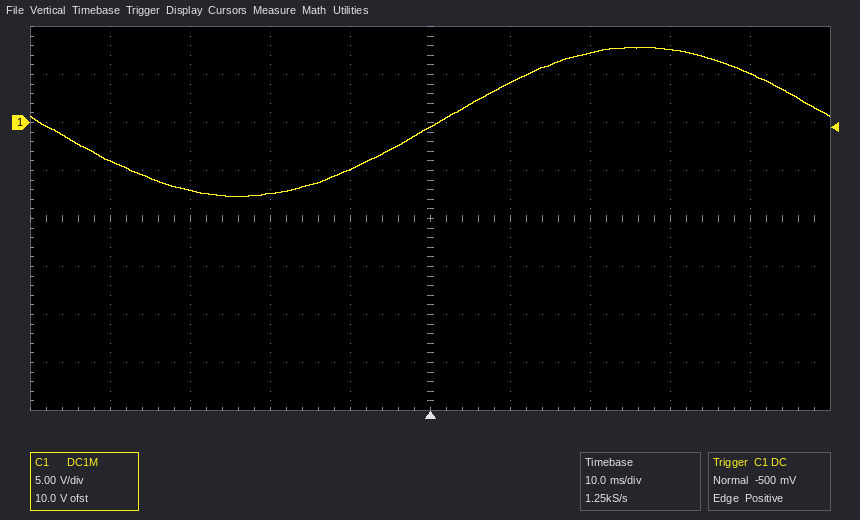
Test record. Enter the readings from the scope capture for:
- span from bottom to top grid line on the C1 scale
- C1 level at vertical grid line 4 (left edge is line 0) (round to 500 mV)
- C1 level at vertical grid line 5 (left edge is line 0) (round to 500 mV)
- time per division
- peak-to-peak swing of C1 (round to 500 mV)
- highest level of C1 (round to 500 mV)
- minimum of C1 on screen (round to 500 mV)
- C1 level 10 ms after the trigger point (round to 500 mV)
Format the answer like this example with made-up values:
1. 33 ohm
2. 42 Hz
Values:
1. 40 V
2. -5.0 V
3. -500 mV
4. 10 ms
5. 15.5 V
6. 8.0 V
7. -7.5 V
8. 4.0 V
